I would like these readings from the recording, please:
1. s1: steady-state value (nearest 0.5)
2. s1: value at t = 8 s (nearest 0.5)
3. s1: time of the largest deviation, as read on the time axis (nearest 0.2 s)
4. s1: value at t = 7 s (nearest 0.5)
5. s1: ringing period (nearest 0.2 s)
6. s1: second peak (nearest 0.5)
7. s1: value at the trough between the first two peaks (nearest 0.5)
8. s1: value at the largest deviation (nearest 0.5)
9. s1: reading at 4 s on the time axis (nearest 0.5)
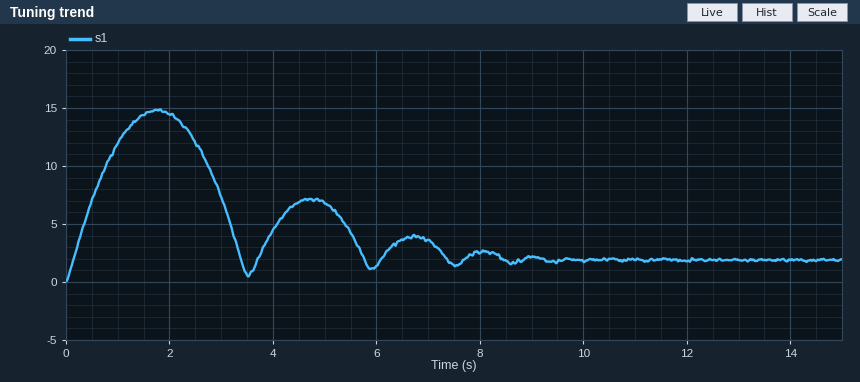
2.0
2.5
1.8 s
3.5
3.0 s
7.0
0.5
15.0
4.5
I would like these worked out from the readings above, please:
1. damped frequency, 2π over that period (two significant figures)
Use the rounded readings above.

2.1 rad/s
